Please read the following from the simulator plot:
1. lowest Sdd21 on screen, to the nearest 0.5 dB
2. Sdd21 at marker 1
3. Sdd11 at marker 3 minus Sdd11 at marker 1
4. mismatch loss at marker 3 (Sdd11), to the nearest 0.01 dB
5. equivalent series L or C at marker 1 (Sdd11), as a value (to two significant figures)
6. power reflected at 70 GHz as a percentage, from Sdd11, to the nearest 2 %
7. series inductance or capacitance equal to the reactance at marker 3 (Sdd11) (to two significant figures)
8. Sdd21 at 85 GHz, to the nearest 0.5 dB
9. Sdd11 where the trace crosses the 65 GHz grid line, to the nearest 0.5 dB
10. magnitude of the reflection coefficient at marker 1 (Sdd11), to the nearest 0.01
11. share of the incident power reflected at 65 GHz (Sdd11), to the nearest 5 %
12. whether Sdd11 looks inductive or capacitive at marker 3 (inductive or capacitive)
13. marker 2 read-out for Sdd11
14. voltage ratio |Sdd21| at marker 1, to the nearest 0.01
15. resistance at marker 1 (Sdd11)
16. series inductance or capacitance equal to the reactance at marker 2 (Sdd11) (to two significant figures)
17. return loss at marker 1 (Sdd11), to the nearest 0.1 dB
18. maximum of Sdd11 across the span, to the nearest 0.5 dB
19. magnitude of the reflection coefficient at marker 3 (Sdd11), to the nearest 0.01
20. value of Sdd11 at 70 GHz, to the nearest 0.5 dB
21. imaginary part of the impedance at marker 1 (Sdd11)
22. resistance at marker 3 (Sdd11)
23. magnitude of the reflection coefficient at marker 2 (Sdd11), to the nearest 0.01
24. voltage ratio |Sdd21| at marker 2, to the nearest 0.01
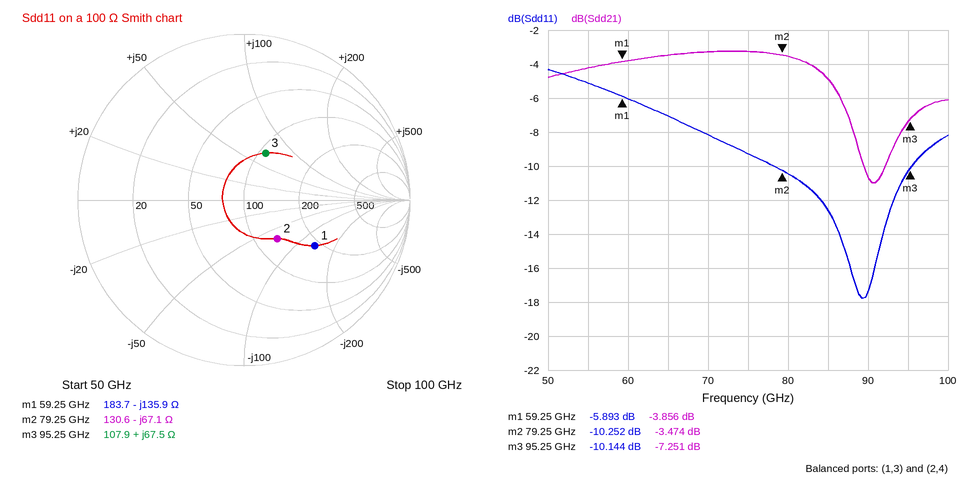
-11.0 dB
-3.856 dB
-4.251 dB
0.44 dB
20 fF
16 %
110 pH
-5.0 dB
-7.0 dB
0.51
20 %
inductive
-10.252 dB
0.64
183.7 Ω
30 fF
5.9 dB
-4.5 dB
0.31
-8.0 dB
-135.9 Ω
107.9 Ω
0.31
0.67
